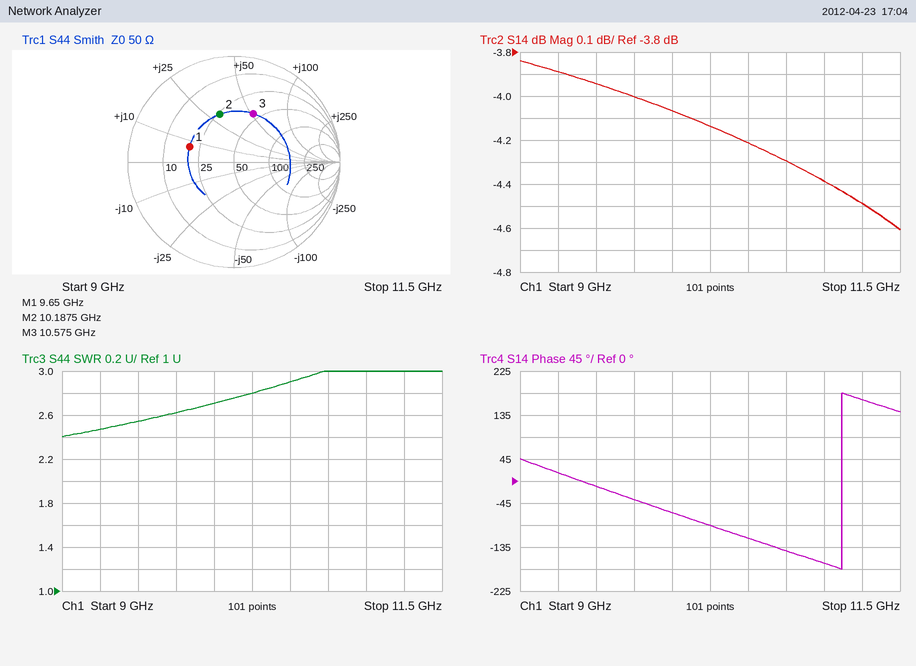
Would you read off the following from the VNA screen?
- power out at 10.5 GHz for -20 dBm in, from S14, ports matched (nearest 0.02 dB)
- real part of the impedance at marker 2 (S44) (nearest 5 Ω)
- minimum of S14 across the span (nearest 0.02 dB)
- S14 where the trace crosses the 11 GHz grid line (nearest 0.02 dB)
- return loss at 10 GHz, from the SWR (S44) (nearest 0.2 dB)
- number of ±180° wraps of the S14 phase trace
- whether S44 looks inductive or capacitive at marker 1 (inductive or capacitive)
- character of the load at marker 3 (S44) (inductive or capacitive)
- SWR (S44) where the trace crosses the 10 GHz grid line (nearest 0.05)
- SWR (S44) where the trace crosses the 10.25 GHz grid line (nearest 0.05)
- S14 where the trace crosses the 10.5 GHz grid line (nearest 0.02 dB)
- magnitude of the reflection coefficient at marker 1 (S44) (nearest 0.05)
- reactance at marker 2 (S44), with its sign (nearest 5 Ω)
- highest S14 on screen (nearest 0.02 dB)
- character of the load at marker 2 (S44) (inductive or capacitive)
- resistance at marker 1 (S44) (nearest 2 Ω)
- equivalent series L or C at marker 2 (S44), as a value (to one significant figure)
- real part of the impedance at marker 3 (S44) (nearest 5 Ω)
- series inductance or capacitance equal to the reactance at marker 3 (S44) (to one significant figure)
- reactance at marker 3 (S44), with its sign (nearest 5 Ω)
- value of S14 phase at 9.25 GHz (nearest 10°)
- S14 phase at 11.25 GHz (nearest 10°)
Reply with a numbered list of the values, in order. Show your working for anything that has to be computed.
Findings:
1. -20 dBm + (-4.22 dB) = -24.22 dBm
2. 25 Ω
3. -4.60 dB
4. -4.38 dB
5. −20 log10((2.7 − 1)/(2.7 + 1)) ≈ 6.8 dB
6. 1
7. inductive
8. inductive
9. 2.70
10. 2.80
11. -4.22 dB
12. 0.45
13. +30 Ω
14. -3.84 dB
15. inductive
16. 20 Ω
17. L = 30 Ω/(2π × 10.1875 GHz) ≈ 469 pH, so 500 pH to one significant figure
18. 45 Ω
19. L = 50 Ω/(2π × 10.575 GHz) ≈ 753 pH, so 800 pH to one significant figure
20. +50 Ω
21. 20°
22. 170°
